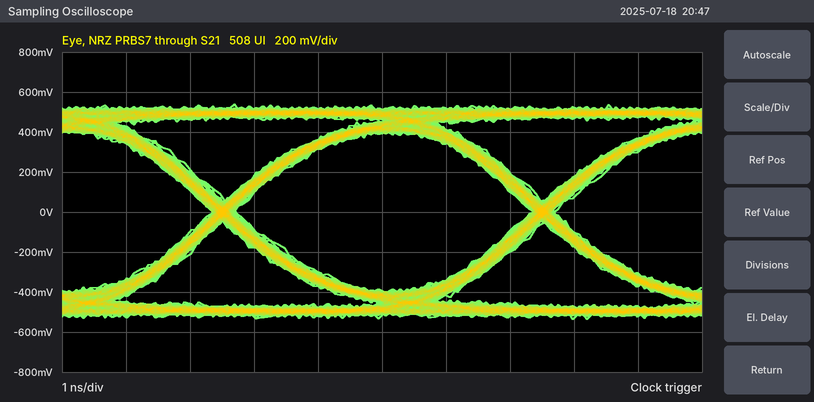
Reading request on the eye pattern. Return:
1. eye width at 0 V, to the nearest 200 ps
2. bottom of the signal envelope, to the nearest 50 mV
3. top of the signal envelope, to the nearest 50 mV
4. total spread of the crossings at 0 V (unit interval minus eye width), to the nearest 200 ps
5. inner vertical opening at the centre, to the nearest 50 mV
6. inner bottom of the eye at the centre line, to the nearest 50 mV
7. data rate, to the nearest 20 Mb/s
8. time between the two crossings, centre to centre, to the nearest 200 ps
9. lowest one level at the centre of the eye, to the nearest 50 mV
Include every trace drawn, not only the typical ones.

4.6 ns
-550 mV
550 mV
400 ps
800 mV
-400 mV
200 Mb/s
5.0 ns
400 mV
